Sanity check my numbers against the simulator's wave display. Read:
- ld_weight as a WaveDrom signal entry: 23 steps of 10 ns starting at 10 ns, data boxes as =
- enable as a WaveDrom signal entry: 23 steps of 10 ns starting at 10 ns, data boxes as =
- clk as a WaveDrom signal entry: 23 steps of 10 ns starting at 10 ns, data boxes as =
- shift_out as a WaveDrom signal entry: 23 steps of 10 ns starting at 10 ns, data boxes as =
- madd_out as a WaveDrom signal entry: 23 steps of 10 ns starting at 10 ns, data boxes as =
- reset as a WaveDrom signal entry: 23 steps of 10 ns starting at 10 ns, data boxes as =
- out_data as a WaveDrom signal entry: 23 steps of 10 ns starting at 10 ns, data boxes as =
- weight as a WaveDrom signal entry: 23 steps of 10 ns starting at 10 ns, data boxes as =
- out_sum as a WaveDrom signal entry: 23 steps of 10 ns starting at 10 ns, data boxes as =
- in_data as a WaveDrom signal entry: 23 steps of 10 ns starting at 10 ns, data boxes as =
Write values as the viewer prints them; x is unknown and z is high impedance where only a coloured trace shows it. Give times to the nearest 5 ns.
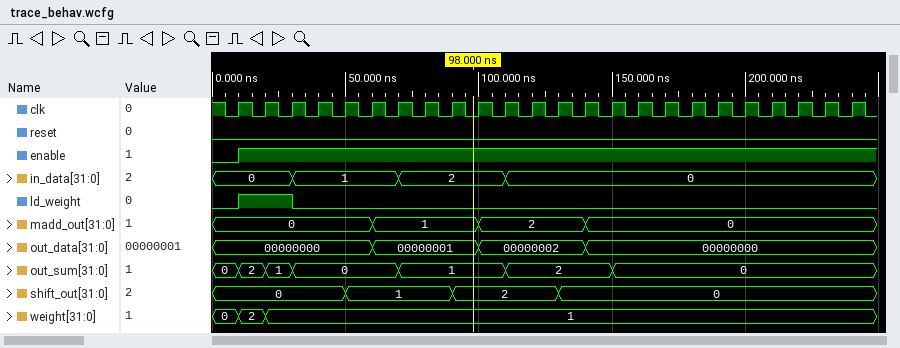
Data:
{name: 'ld_weight', wave: '1.0....................'}
{name: 'enable', wave: '1......................'}
{name: 'clk', wave: 'p......................'}
{name: 'shift_out', wave: '=...=...=...=..........', data: '0 1 2 0'}
{name: 'madd_out', wave: '=....=...=...=.........', data: '0 1 2 0'}
{name: 'reset', wave: '0......................'}
{name: 'out_data', wave: '=....=...=...=.........', data: '00000000 00000001 00000002 00000000'}
{name: 'weight', wave: '==.....................', data: '2 1'}
{name: 'out_sum', wave: '===...=...=...=........', data: '2 1 0 1 2 0'}
{name: 'in_data', wave: '=.=...=...=............', data: '0 1 2 0'}
